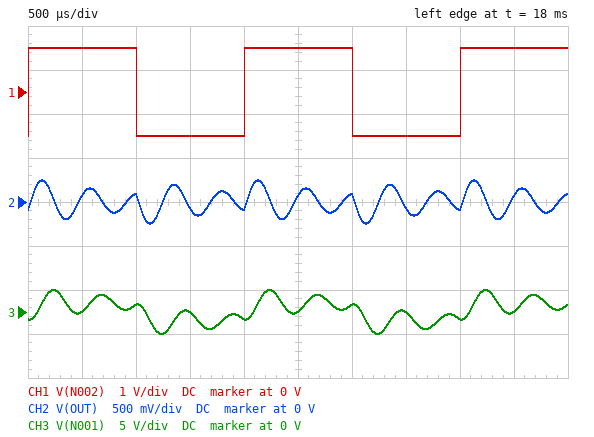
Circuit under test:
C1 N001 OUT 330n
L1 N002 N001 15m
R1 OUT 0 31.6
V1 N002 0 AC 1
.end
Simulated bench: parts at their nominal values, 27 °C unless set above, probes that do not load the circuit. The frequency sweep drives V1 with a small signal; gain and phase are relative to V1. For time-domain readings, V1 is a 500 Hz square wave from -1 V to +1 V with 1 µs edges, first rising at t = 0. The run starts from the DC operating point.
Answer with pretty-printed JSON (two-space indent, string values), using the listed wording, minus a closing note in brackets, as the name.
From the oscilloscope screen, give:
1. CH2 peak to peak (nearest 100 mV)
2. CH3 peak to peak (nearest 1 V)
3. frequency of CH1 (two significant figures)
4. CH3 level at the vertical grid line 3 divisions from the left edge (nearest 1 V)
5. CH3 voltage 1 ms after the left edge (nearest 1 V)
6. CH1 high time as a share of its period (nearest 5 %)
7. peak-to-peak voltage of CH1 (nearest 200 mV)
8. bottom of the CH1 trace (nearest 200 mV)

{
  "CH2 peak to peak": "500 mV",
  "CH3 peak to peak": "5 V",
  "frequency of CH1": "500 Hz",
  "CH3 level at the vertical grid line 3 divisions from the left edge": "0 V",
  "CH3 voltage 1 ms after the left edge": "1 V",
  "CH1 high time as a share of its period": "50 %",
  "peak-to-peak voltage of CH1": "2.0 V",
  "bottom of the CH1 trace": "-1.0 V"
}
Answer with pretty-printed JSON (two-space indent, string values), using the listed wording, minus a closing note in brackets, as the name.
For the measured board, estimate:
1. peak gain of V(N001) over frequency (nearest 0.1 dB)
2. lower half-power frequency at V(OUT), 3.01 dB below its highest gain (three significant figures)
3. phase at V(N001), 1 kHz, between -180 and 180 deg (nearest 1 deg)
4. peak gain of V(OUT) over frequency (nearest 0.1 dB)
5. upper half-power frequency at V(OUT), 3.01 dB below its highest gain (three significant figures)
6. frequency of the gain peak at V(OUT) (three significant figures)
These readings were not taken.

{
  "peak gain of V(N001) over frequency": "16.7 dB",
  "lower half-power frequency at V(OUT), 3.01 dB below its highest gain": "2.10 kHz",
  "phase at V(N001), 1 kHz, between -180 and 180 deg": "-1 deg",
  "peak gain of V(OUT) over frequency": "0 dB",
  "upper half-power frequency at V(OUT), 3.01 dB below its highest gain": "2.44 kHz",
  "frequency of the gain peak at V(OUT)": "2.26 kHz"
}
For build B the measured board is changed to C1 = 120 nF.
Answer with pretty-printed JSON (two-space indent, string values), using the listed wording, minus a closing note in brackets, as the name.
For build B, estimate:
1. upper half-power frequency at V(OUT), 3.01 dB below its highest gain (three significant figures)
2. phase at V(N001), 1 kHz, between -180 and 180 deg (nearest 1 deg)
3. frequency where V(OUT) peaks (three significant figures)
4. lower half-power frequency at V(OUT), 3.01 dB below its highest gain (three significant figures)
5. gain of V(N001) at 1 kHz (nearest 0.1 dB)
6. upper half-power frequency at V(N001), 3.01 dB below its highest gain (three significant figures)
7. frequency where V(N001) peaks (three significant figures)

{
  "upper half-power frequency at V(OUT), 3.01 dB below its highest gain": "3.92 kHz",
  "phase at V(N001), 1 kHz, between -180 and 180 deg": "0 deg",
  "frequency where V(OUT) peaks": "3.75 kHz",
  "lower half-power frequency at V(OUT), 3.01 dB below its highest gain": "3.59 kHz",
  "gain of V(N001) at 1 kHz": "0.6 dB",
  "upper half-power frequency at V(N001), 3.01 dB below its highest gain": "3.91 kHz",
  "frequency where V(N001) peaks": "3.74 kHz"
}
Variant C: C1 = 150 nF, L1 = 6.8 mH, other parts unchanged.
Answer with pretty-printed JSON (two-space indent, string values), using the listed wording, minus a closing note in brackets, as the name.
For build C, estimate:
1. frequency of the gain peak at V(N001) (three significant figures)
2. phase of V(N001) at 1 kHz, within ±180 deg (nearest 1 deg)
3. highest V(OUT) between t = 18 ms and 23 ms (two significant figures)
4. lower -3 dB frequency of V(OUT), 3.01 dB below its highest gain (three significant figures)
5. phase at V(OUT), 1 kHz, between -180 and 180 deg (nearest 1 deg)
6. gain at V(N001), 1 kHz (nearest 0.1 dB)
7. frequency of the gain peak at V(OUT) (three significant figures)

{
  "frequency of the gain peak at V(N001)": "4.96 kHz",
  "phase of V(N001) at 1 kHz, within ±180 deg": "0 deg",
  "highest V(OUT) between t = 18 ms and 23 ms": "240 mV",
  "lower -3 dB frequency of V(OUT), 3.01 dB below its highest gain": "4.63 kHz",
  "phase at V(OUT), 1 kHz, between -180 and 180 deg": "88 deg",
  "gain at V(N001), 1 kHz": "0.4 dB",
  "frequency of the gain peak at V(OUT)": "4.98 kHz"
}
